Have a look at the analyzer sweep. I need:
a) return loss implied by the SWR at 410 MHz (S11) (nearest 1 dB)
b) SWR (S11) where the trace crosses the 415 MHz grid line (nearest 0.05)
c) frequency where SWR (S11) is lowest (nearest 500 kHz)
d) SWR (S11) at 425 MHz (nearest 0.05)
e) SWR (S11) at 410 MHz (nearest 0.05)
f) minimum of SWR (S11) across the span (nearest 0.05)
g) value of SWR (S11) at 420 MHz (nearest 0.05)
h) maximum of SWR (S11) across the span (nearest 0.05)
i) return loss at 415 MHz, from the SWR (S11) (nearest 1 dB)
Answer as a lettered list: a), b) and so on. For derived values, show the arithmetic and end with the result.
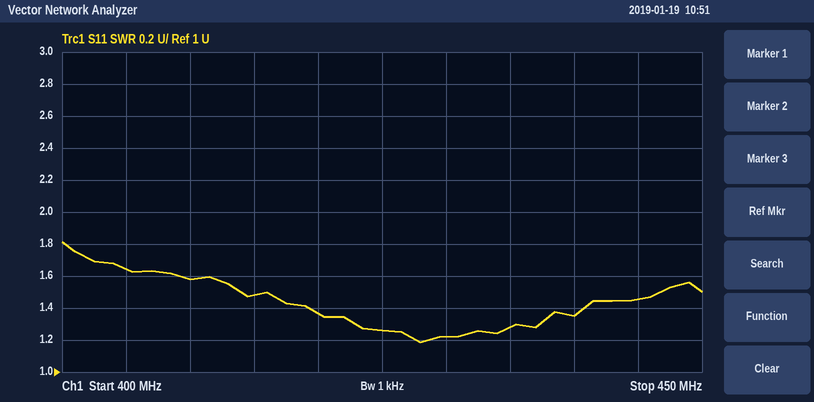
a) −20 log10((1.6 − 1)/(1.6 + 1)) ≈ 13 dB
b) 1.50
c) 428.0 MHz
d) 1.25
e) 1.60
f) 1.20
g) 1.35
h) 1.80
i) −20 log10((1.5 − 1)/(1.5 + 1)) ≈ 14 dB
